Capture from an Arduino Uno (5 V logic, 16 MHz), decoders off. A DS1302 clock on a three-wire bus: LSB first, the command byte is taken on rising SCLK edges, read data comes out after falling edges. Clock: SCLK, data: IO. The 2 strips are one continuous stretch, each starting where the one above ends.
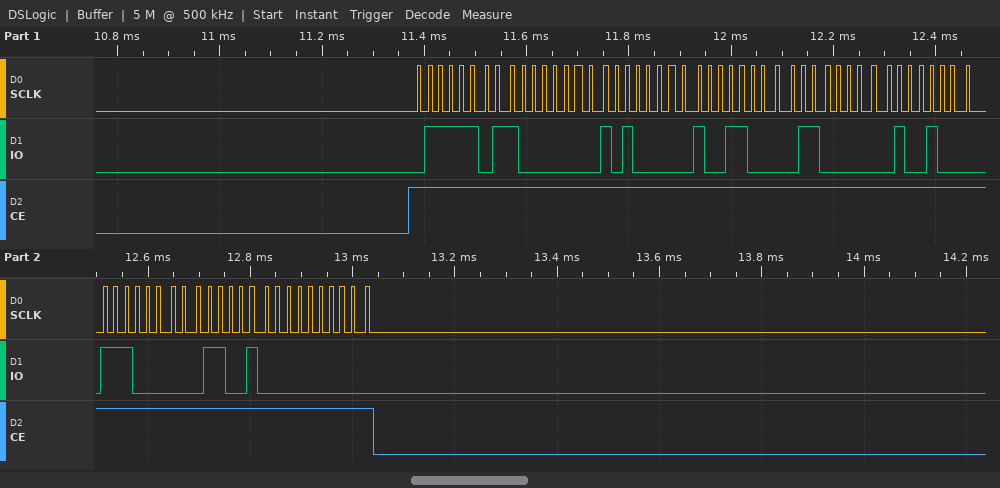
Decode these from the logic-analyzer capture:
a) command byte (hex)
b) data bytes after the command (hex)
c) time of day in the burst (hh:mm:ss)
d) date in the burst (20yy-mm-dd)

0xBE
01 05 19 06 12 07 26 00
19:05:01
2026-12-06
